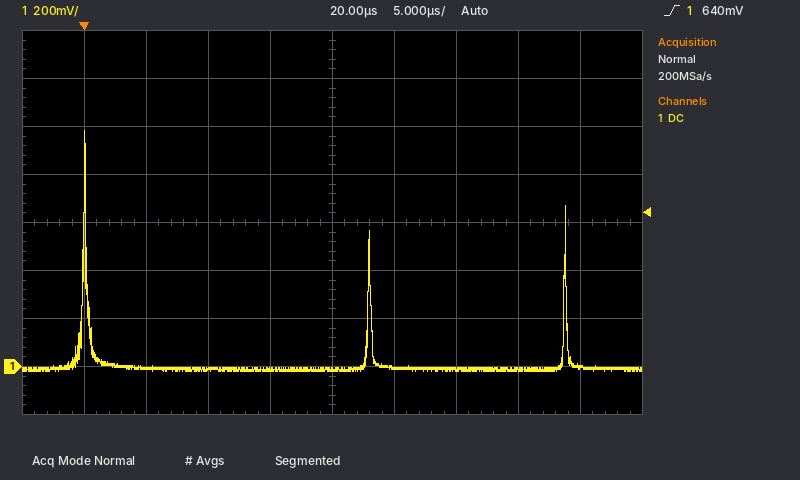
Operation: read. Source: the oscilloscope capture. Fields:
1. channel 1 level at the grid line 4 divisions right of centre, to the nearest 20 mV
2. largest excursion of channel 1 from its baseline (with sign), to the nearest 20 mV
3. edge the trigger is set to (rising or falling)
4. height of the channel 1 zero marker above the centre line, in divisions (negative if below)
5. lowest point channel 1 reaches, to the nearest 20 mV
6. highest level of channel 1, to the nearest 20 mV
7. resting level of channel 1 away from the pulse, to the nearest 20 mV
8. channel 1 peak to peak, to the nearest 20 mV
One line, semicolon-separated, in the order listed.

0 mV; +1.00 V; rising; -3.0 div; -20 mV; 980 mV; -20 mV; 1.00 V
